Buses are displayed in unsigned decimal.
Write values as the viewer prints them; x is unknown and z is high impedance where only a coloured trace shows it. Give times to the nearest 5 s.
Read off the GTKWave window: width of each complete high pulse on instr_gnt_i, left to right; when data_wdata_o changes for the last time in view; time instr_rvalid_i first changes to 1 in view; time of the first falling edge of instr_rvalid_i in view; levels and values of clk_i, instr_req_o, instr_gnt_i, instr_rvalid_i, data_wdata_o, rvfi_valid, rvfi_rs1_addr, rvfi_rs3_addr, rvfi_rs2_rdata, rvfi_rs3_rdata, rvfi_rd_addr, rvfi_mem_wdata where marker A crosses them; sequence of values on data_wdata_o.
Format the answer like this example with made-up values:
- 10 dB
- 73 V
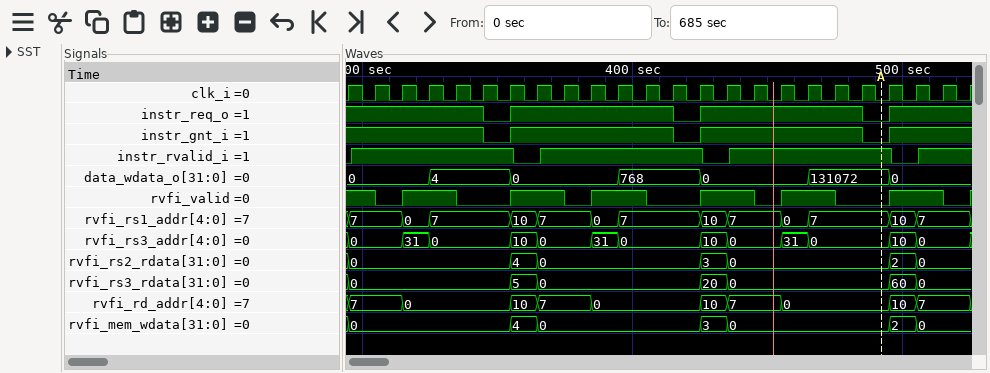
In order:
- 60 s, 60 s
- 495 s
- 295 s
- 355 s
- clk_i=0, instr_req_o=0, instr_gnt_i=0, instr_rvalid_i=1, data_wdata_o=131072, rvfi_valid=0, rvfi_rs1_addr=7, rvfi_rs3_addr=0, rvfi_rs2_rdata=0, rvfi_rs3_rdata=0, rvfi_rd_addr=0, rvfi_mem_wdata=0
- 0, 4, 0, 768, 0, 131072, 0
